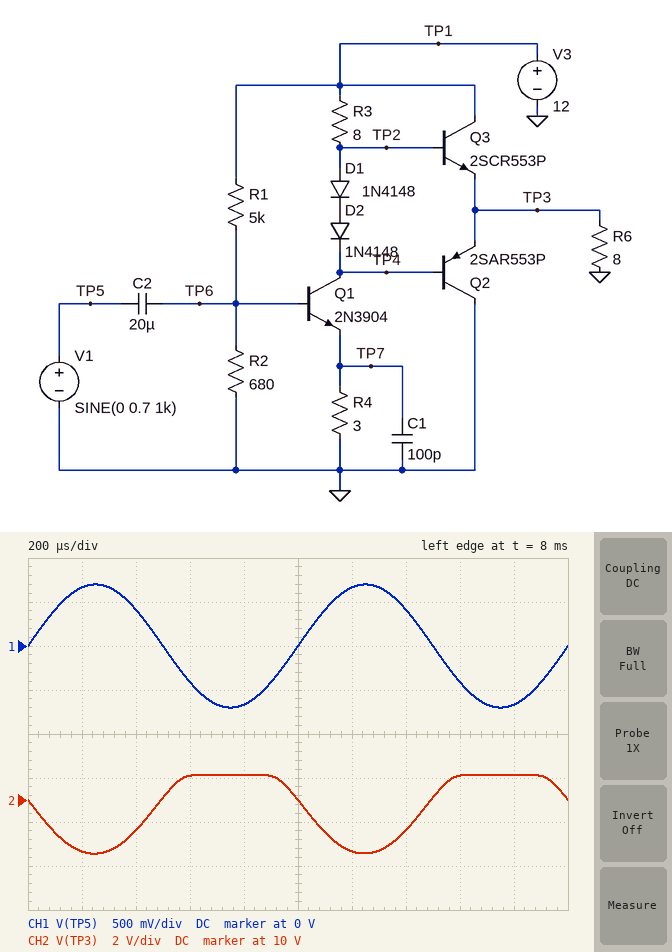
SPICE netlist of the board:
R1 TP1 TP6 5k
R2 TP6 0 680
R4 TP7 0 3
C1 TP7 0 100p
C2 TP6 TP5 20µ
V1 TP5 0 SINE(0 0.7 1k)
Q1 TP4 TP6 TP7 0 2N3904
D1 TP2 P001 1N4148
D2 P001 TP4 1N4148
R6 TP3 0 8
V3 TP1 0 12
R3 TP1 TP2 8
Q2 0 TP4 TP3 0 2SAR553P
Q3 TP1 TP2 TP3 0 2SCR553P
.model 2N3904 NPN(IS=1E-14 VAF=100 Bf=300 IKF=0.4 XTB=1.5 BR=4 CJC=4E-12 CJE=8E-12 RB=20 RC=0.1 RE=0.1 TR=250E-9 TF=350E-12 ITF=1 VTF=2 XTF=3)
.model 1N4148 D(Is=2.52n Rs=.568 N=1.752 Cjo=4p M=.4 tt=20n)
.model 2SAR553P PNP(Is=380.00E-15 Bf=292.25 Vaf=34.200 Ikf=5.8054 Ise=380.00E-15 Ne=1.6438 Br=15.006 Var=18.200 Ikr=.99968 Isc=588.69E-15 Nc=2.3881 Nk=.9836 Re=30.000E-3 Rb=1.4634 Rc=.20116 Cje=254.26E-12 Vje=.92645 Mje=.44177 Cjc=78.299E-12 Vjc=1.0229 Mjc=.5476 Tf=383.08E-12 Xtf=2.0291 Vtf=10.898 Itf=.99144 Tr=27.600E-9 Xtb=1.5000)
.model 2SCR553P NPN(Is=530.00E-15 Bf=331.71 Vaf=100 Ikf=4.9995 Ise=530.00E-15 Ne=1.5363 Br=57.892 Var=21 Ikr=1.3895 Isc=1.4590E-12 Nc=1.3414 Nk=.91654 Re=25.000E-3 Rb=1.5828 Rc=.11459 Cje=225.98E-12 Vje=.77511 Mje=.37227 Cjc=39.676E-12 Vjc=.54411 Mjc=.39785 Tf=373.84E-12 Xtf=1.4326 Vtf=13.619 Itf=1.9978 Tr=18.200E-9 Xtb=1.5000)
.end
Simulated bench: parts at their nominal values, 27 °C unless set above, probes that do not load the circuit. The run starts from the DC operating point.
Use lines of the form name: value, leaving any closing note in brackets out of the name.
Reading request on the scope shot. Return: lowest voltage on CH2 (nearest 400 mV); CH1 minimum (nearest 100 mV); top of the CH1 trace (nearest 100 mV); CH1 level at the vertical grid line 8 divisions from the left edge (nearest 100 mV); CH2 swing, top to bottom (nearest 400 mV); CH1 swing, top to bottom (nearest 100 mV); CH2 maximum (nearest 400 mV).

lowest voltage on CH2: 7.6 V
CH1 minimum: -700 mV
top of the CH1 trace: 700 mV
CH1 level at the vertical grid line 8 divisions from the left edge: -400 mV
CH2 swing, top to bottom: 3.6 V
CH1 swing, top to bottom: 1.4 V
CH2 maximum: 11.2 V
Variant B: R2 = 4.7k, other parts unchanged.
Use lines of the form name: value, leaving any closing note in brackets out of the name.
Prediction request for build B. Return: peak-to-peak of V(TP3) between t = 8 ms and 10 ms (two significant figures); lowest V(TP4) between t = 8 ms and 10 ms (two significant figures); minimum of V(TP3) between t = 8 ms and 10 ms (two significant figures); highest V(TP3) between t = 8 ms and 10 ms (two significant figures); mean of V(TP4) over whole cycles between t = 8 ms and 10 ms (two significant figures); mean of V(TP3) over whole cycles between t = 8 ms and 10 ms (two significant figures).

peak-to-peak of V(TP3) between t = 8 ms and 10 ms: 4.5 V
lowest V(TP4) between t = 8 ms and 10 ms: 4.8 V
minimum of V(TP3) between t = 8 ms and 10 ms: 5.7 V
highest V(TP3) between t = 8 ms and 10 ms: 10 V
mean of V(TP4) over whole cycles between t = 8 ms and 10 ms: 7.0 V
mean of V(TP3) over whole cycles between t = 8 ms and 10 ms: 7.9 V
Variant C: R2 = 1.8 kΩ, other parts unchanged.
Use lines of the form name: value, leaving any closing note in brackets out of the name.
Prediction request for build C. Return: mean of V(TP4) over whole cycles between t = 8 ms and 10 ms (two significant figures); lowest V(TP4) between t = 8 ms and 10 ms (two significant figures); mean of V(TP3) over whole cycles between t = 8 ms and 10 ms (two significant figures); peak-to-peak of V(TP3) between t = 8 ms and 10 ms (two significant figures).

mean of V(TP4) over whole cycles between t = 8 ms and 10 ms: 7.7 V
lowest V(TP4) between t = 8 ms and 10 ms: 5.3 V
mean of V(TP3) over whole cycles between t = 8 ms and 10 ms: 8.5 V
peak-to-peak of V(TP3) between t = 8 ms and 10 ms: 4.6 V
